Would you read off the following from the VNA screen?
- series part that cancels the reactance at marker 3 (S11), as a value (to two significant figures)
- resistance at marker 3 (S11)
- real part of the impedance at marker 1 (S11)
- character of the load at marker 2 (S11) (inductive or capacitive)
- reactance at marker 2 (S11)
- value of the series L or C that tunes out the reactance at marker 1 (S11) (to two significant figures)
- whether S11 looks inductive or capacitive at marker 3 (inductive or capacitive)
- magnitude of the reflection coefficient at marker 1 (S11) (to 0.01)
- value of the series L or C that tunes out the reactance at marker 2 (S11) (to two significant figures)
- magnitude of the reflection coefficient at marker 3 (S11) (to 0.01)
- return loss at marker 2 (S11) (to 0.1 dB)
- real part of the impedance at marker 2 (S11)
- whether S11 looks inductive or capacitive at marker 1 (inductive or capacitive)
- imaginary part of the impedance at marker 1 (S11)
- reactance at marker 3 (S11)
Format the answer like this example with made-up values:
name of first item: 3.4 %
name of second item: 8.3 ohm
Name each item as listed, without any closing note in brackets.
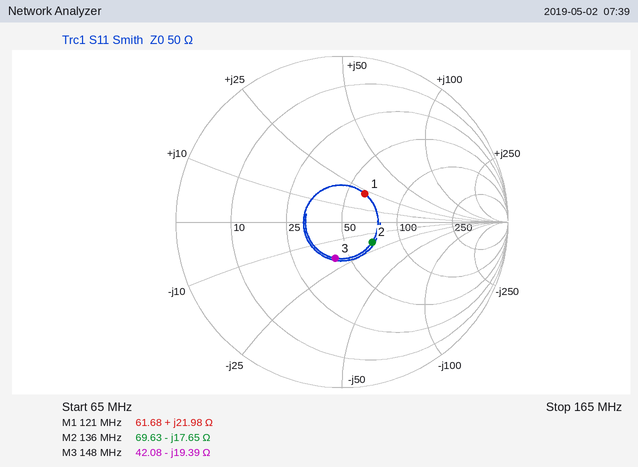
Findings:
series part that cancels the reactance at marker 3 (S11), as a value: 21 nH
resistance at marker 3: 42.08 Ω
real part of the impedance at marker 1: 61.68 Ω
character of the load at marker 2 (S11): capacitive
reactance at marker 2: -17.65 Ω
value of the series L or C that tunes out the reactance at marker 1 (S11): 60 pF
whether S11 looks inductive or capacitive at marker 3: capacitive
magnitude of the reflection coefficient at marker 1 (S11): 0.22
value of the series L or C that tunes out the reactance at marker 2 (S11): 21 nH
magnitude of the reflection coefficient at marker 3 (S11): 0.22
return loss at marker 2 (S11): 13.2 dB
real part of the impedance at marker 2: 69.63 Ω
whether S11 looks inductive or capacitive at marker 1: inductive
imaginary part of the impedance at marker 1: +21.98 Ω
reactance at marker 3: -19.39 Ω
